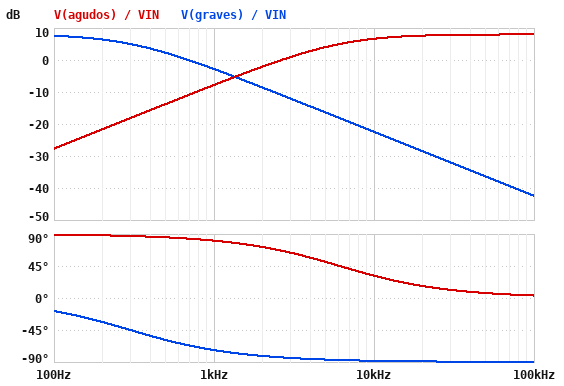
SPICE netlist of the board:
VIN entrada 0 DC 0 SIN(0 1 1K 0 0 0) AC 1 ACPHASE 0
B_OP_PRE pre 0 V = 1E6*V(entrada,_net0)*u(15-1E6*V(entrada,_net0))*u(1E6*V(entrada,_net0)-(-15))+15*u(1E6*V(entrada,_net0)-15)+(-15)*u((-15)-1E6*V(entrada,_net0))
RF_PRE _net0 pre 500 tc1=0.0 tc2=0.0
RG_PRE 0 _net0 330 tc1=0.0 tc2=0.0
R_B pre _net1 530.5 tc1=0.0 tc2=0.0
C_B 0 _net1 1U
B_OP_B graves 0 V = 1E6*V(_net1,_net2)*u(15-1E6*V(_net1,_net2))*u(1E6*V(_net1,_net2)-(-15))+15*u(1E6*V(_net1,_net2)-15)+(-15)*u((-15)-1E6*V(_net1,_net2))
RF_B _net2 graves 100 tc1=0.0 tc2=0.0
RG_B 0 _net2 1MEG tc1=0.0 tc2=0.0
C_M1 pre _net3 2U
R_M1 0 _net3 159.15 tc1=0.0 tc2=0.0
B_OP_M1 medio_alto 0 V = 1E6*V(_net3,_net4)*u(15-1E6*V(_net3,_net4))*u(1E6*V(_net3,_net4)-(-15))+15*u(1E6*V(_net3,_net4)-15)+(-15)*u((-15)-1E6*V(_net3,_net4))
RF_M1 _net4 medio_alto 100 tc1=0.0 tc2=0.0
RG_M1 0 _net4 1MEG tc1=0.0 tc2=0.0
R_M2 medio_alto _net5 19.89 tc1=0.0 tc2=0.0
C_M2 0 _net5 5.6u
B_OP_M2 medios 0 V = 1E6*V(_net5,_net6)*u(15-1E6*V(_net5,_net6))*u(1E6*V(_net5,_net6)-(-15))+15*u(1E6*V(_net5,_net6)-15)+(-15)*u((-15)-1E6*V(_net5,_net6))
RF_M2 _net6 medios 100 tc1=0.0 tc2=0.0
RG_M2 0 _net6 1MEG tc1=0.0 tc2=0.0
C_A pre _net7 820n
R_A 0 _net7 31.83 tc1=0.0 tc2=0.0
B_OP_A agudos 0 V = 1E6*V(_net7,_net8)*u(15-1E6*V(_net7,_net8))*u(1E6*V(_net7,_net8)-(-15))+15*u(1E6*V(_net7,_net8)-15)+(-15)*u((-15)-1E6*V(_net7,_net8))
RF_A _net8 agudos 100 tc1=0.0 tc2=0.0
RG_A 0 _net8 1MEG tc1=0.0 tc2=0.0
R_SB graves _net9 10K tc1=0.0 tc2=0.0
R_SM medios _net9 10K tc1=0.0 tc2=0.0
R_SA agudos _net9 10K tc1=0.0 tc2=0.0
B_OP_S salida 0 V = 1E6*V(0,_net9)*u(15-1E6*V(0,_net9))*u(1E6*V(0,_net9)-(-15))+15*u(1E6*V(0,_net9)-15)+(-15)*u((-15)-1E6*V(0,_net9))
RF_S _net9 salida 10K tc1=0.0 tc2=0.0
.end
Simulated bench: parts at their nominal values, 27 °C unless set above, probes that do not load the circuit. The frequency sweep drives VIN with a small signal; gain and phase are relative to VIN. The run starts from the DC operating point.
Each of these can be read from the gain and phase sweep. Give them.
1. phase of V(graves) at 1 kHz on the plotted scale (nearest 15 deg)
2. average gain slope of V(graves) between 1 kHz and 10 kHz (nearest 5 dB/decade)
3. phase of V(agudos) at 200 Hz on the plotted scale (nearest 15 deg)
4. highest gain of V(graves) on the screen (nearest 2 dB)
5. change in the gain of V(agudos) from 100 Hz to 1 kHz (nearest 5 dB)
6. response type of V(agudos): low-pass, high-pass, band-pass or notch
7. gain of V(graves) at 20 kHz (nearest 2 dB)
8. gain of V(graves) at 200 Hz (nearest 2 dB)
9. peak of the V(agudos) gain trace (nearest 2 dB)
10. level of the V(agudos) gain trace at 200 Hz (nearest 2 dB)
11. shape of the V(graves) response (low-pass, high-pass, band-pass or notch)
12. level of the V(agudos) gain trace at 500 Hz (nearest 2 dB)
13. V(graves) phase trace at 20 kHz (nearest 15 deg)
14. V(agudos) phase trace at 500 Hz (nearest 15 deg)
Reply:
-75 deg
-20 dB/decade
90 deg
8 dB
20 dB
high-pass
-28 dB
6 dB
8 dB
-22 dB
low-pass
-14 dB
-90 deg
90 deg
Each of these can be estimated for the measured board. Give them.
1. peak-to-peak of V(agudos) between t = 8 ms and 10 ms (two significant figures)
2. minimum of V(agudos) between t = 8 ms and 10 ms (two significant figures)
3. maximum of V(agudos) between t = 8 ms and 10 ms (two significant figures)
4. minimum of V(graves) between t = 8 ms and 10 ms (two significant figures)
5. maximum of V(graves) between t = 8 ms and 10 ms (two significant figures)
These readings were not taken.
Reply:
810 mV
-410 mV
410 mV
-720 mV
720 mV
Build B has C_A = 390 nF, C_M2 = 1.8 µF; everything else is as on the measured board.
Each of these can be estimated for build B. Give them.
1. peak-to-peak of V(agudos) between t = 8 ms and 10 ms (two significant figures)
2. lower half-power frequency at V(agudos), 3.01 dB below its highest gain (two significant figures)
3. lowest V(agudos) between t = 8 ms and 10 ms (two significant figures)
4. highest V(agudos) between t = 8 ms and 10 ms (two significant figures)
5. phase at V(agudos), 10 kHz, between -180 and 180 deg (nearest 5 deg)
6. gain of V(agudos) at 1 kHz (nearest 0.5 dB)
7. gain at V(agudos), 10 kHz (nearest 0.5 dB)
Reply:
390 mV
13 kHz
-200 mV
200 mV
50 deg
-14.0 dB
4.0 dB
